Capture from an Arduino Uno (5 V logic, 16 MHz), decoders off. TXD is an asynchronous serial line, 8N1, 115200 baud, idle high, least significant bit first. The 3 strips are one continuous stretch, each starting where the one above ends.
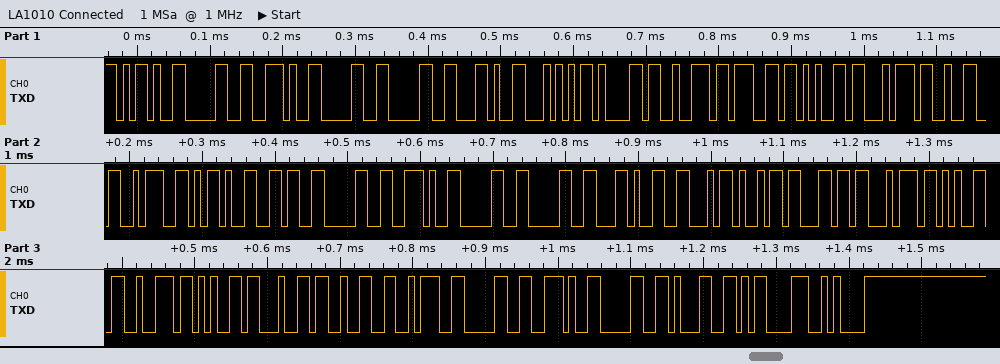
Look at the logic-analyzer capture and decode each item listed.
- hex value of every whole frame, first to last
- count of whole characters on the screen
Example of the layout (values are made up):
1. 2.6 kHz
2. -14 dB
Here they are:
1. 0x2D 0x30 0x2E 0x30 0x30 0x2C 0x54 0x61 0x72 0x67 0x65 0x74 0x32 0x3A 0x2D 0x36 0x30 0x2E 0x30 0x30 0x2C 0x46 0x69 0x6C 0x74 0x65 0x72 0x65 0x64 0x32 0x3A 0x30 0x2E 0x30 0x31 0x0D 0x0A
2. 37
